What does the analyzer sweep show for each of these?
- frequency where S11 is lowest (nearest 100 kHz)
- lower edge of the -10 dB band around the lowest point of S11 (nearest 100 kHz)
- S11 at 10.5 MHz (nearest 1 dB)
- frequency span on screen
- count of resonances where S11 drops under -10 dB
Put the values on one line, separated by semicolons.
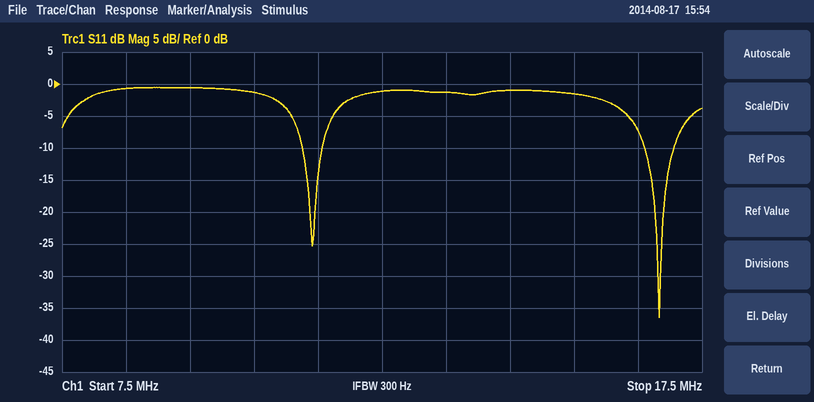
16.8 MHz; 16.6 MHz; -1 dB; 10 MHz; 2
